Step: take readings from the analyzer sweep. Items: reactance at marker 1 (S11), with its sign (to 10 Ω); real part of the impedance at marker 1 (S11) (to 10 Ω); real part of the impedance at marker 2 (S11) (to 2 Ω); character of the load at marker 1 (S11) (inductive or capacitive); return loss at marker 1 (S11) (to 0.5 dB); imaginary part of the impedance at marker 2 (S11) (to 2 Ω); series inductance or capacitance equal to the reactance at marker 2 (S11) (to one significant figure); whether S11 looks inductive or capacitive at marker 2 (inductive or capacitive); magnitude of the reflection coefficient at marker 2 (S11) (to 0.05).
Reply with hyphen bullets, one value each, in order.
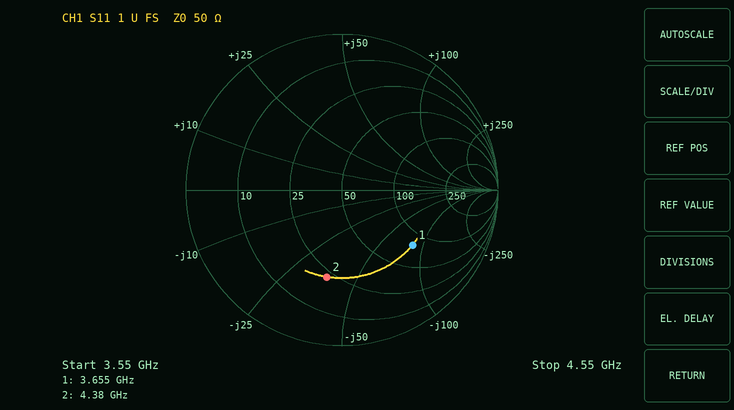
- -80 Ω
- 80 Ω
- 22 Ω
- capacitive
- 5.0 dB
- -36 Ω
- 1.0 pF
- capacitive
- 0.55
